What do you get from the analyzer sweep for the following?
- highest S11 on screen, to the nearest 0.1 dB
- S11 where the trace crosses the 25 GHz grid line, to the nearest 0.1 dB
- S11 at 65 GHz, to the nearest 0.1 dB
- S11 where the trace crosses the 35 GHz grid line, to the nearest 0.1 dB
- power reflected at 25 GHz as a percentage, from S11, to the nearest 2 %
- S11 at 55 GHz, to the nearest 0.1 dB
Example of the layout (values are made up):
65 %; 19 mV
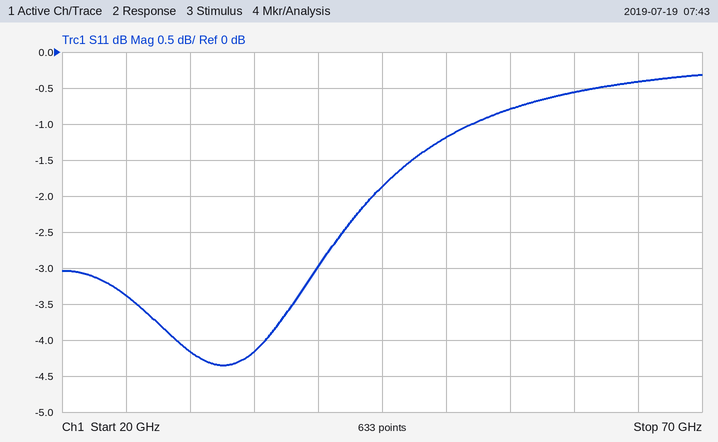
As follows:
-0.3 dB; -3.4 dB; -0.4 dB; -4.2 dB; 46 %; -0.8 dB
